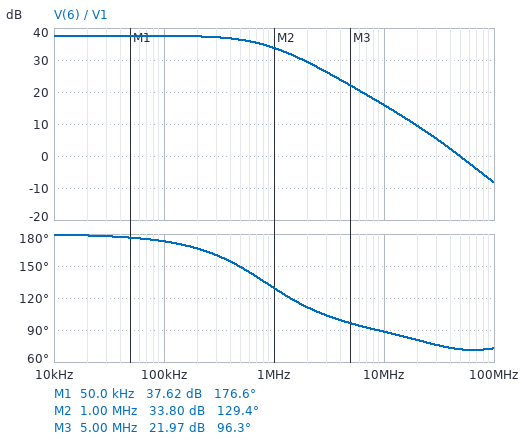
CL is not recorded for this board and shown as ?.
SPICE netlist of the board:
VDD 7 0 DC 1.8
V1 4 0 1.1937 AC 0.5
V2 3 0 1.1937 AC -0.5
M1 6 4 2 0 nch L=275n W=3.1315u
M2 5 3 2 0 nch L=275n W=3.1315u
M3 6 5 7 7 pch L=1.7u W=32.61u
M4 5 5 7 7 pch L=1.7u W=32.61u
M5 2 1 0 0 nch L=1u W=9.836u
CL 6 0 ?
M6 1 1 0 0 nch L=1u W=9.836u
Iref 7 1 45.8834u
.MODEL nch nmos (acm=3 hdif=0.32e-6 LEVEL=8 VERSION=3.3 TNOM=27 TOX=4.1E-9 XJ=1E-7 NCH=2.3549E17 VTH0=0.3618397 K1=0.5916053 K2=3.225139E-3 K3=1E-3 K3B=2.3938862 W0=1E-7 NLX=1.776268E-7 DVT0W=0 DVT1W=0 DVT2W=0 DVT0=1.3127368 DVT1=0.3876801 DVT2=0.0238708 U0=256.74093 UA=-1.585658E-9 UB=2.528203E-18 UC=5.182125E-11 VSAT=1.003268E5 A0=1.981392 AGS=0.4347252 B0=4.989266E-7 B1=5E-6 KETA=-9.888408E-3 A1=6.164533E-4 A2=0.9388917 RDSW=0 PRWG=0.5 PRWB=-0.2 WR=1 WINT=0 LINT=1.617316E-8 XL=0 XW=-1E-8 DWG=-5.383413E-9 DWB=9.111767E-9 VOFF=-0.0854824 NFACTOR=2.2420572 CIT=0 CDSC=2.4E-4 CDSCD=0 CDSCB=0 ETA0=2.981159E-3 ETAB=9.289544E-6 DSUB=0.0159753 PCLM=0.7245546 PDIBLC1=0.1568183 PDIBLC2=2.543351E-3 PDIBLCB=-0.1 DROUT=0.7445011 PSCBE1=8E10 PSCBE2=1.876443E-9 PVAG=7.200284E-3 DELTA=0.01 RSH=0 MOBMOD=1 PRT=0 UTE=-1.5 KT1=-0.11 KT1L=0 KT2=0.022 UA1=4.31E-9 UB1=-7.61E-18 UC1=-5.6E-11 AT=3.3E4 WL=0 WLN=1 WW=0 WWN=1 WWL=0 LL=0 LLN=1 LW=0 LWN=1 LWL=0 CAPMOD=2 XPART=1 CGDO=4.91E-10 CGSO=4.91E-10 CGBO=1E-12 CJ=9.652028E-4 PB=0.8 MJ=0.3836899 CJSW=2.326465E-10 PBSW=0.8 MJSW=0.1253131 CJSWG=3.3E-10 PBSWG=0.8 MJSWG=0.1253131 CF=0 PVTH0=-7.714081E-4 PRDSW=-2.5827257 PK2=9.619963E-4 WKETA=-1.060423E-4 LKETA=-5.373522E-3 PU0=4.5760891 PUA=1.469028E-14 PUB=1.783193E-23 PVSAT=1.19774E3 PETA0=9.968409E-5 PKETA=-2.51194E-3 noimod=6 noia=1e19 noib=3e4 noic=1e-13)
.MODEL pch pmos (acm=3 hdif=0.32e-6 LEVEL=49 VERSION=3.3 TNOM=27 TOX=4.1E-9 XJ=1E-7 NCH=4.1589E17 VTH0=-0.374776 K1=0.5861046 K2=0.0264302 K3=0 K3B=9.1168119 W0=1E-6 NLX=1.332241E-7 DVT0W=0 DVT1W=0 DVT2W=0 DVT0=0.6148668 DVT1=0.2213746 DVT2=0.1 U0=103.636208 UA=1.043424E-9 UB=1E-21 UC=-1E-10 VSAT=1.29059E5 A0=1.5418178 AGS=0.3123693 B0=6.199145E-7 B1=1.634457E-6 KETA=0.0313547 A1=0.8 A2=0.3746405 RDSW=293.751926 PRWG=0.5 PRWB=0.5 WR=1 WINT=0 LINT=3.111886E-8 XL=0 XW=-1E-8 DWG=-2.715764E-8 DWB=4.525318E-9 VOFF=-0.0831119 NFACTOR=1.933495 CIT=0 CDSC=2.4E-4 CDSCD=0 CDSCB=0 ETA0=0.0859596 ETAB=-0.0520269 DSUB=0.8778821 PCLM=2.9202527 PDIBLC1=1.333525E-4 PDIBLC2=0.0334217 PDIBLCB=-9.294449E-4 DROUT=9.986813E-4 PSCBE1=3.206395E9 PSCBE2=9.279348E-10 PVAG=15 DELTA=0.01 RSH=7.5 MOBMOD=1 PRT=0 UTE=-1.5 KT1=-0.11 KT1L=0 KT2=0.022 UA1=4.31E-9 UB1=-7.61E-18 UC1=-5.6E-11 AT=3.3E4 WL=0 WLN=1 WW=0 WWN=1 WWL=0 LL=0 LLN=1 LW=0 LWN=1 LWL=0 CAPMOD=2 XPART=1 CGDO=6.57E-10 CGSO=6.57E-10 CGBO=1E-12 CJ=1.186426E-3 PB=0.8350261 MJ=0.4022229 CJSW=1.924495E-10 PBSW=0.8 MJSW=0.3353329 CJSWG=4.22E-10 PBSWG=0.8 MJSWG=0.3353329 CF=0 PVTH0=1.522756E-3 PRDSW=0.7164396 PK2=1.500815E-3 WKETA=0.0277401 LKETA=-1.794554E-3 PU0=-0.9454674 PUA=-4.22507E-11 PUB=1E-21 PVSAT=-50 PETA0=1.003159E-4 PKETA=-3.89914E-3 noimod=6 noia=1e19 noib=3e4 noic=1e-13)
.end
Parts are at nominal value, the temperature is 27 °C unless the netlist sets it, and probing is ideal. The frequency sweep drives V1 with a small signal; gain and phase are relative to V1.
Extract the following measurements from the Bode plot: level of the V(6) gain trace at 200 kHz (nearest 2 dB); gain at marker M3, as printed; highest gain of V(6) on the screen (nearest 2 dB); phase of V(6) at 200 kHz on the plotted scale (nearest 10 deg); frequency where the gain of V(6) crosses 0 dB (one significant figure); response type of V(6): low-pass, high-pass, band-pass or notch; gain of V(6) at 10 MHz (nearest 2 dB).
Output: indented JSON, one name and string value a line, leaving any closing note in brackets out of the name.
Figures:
{
  "level of the V(6) gain trace at 200 kHz": "38 dB",
  "gain at marker M3, as printed": "21.97 dB",
  "highest gain of V(6) on the screen": "38 dB",
  "phase of V(6) at 200 kHz on the plotted scale": "170 deg",
  "frequency where the gain of V(6) crosses 0 dB": "50 MHz",
  "response type of V(6): low-pass, high-pass, band-pass or notch": "low-pass",
  "gain of V(6) at 10 MHz": "16 dB"
}
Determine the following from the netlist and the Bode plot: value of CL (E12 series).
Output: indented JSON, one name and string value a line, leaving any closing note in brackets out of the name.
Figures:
{
  "value of CL": "1.2 pF"
}
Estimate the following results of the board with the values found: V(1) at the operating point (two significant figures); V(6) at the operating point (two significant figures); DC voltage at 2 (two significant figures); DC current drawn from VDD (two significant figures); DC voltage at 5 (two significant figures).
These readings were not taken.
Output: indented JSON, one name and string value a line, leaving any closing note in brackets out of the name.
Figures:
{
  "V(1) at the operating point": "610 mV",
  "V(6) at the operating point": "1.2 V",
  "DC voltage at 2": "490 mV",
  "DC current drawn from VDD": "91 µA",
  "DC voltage at 5": "1.2 V"
}
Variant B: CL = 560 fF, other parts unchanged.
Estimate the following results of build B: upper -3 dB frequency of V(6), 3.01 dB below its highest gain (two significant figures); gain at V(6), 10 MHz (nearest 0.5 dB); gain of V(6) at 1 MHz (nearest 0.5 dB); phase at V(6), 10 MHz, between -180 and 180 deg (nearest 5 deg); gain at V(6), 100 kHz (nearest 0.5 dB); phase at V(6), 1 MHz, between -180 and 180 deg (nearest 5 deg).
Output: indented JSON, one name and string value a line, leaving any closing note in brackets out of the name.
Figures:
{
  "upper -3 dB frequency of V(6), 3.01 dB below its highest gain": "1.7 MHz",
  "gain at V(6), 10 MHz": "22.0 dB",
  "gain of V(6) at 1 MHz": "36.5 dB",
  "phase at V(6), 10 MHz, between -180 and 180 deg": "95 deg",
  "gain at V(6), 100 kHz": "37.5 dB",
  "phase at V(6), 1 MHz, between -180 and 180 deg": "150 deg"
}
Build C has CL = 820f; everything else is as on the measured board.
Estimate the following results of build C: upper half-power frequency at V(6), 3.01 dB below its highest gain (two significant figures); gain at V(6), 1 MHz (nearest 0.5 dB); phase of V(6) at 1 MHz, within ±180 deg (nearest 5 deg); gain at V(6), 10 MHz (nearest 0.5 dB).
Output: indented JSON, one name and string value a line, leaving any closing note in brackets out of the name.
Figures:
{
  "upper half-power frequency at V(6), 3.01 dB below its highest gain": "1.2 MHz",
  "gain at V(6), 1 MHz": "35.5 dB",
  "phase of V(6) at 1 MHz, within ±180 deg": "140 deg",
  "gain at V(6), 10 MHz": "19.0 dB"
}
